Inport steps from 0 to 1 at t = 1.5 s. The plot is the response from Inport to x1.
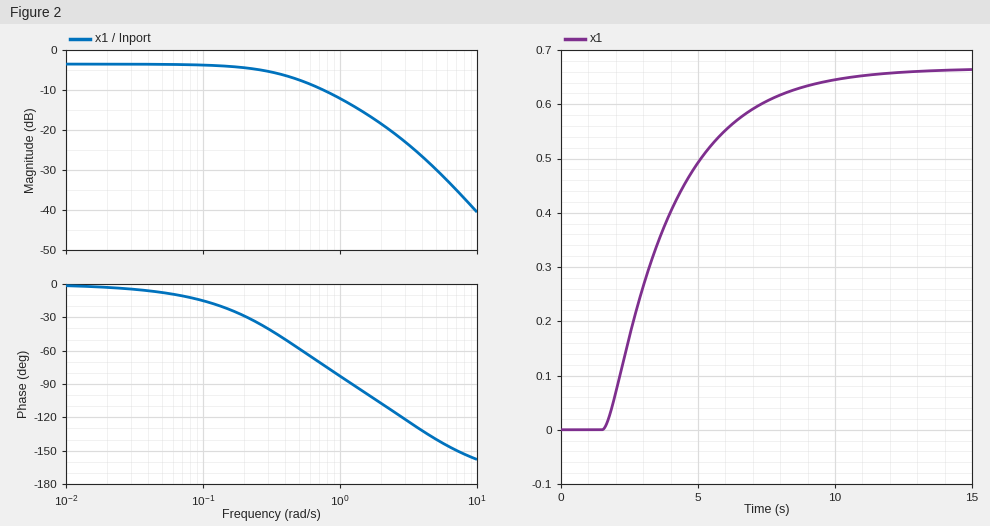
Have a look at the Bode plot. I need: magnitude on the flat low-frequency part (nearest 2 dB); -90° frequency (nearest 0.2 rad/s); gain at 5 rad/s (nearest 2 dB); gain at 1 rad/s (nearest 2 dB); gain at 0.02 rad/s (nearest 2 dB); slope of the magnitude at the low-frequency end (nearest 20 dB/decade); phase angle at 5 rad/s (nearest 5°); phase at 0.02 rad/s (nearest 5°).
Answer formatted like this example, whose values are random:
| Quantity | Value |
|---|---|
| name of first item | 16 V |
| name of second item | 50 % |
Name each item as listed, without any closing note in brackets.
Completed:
| Quantity | Value |
|---|---|
| magnitude on the flat low-frequency part | -4 dB |
| -90° frequency | 1.2 rad/s |
| gain at 5 rad/s | -30 dB |
| gain at 1 rad/s | -12 dB |
| gain at 0.02 rad/s | -4 dB |
| slope of the magnitude at the low-frequency end | 0 dB/decade |
| phase angle at 5 rad/s | -140° |
| phase at 0.02 rad/s | -5° |
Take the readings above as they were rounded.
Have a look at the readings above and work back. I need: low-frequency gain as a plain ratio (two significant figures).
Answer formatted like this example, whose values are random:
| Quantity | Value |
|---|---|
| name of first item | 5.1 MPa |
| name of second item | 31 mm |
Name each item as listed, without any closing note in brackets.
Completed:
| Quantity | Value |
|---|---|
| low-frequency gain as a plain ratio | 0.63 |
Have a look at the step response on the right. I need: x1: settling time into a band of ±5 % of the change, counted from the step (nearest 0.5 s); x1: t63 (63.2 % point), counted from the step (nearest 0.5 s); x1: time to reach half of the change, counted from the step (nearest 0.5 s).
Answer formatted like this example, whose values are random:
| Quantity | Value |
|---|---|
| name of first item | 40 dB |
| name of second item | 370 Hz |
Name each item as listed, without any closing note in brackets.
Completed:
| Quantity | Value |
|---|---|
| x1: settling time into a band of ±5 % of the change, counted from the step | 7.5 s |
| x1: t63 (63.2 % point), counted from the step | 2.5 s |
| x1: time to reach half of the change, counted from the step | 2.0 s |
